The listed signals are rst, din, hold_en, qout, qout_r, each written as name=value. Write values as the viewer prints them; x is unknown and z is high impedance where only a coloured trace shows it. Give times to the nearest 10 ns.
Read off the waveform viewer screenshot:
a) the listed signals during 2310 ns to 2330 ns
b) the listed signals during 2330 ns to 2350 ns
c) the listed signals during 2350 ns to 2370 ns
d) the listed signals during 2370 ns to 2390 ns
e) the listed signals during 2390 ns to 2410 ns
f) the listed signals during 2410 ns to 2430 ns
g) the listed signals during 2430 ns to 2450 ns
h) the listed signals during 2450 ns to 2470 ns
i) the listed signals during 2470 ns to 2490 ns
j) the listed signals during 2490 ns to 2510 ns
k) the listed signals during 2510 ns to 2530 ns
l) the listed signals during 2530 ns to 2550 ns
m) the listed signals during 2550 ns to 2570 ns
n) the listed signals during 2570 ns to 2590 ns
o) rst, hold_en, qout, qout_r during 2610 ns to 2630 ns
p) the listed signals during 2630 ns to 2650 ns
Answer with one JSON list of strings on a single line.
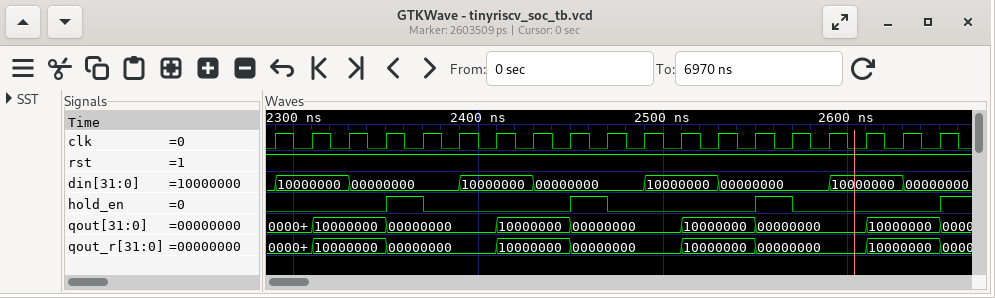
["rst=1, din=10000000, hold_en=0, qout=10000000, qout_r=10000000", "rst=1, din=00000000, hold_en=0, qout=10000000, qout_r=10000000", "rst=1, din=00000000, hold_en=1, qout=00000000, qout_r=00000000", "rst=1, din=00000000, hold_en=0, qout=00000000, qout_r=00000000", "rst=1, din=10000000, hold_en=0, qout=00000000, qout_r=00000000", "rst=1, din=10000000, hold_en=0, qout=10000000, qout_r=10000000", "rst=1, din=00000000, hold_en=0, qout=10000000, qout_r=10000000", "rst=1, din=00000000, hold_en=1, qout=00000000, qout_r=00000000", "rst=1, din=00000000, hold_en=0, qout=00000000, qout_r=00000000", "rst=1, din=10000000, hold_en=0, qout=00000000, qout_r=00000000", "rst=1, din=10000000, hold_en=0, qout=10000000, qout_r=10000000", "rst=1, din=00000000, hold_en=0, qout=10000000, qout_r=10000000", "rst=1, din=00000000, hold_en=1, qout=00000000, qout_r=00000000", "rst=1, din=00000000, hold_en=0, qout=00000000, qout_r=00000000", "rst=1, hold_en=0, qout=10000000, qout_r=10000000", "rst=1, din=00000000, hold_en=0, qout=10000000, qout_r=10000000"]
